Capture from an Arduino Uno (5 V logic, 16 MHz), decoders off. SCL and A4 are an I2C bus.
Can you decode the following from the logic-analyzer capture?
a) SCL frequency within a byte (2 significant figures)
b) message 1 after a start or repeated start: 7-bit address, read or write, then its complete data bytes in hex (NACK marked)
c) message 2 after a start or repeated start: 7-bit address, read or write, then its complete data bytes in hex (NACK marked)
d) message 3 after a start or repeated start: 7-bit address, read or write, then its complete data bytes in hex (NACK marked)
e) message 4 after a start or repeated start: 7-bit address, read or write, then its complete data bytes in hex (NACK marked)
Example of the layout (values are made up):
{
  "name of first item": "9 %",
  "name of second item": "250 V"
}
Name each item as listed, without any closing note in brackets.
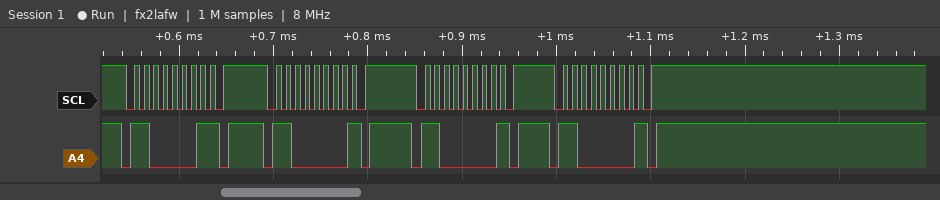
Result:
{
  "SCL frequency within a byte": "100 kHz",
  "message 1 after a start or repeated start: 7-bit address, read or write, then its complete data bytes in hex": "0x60 read NACK",
  "message 2 after a start or repeated start: 7-bit address, read or write, then its complete data bytes in hex": "0x60 write NACK",
  "message 3 after a start or repeated start: 7-bit address, read or write, then its complete data bytes in hex": "0x60 write NACK",
  "message 4 after a start or repeated start: 7-bit address, read or write, then its complete data bytes in hex": "0x60 write NACK"
}
